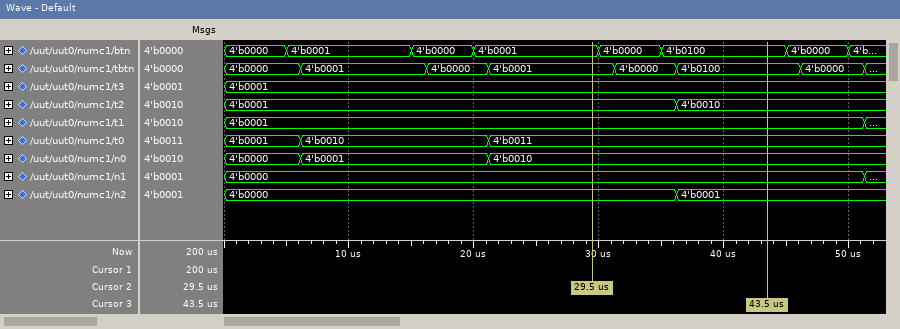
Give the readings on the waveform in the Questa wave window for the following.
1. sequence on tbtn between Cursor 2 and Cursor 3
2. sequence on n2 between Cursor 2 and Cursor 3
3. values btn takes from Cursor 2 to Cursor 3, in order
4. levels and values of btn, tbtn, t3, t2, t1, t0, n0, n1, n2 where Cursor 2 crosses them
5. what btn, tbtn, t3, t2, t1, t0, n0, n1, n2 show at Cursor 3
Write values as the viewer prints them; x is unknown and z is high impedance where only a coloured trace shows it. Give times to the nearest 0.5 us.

4'b0001, 4'b0000, 4'b0100
4'b0000, 4'b0001
4'b0001, 4'b0000, 4'b0100
btn=4'b0001, tbtn=4'b0001, t3=4'b0001, t2=4'b0001, t1=4'b0001, t0=4'b0011, n0=4'b0010, n1=4'b0000, n2=4'b0000
btn=4'b0100, tbtn=4'b0100, t3=4'b0001, t2=4'b0010, t1=4'b0001, t0=4'b0011, n0=4'b0010, n1=4'b0000, n2=4'b0001
